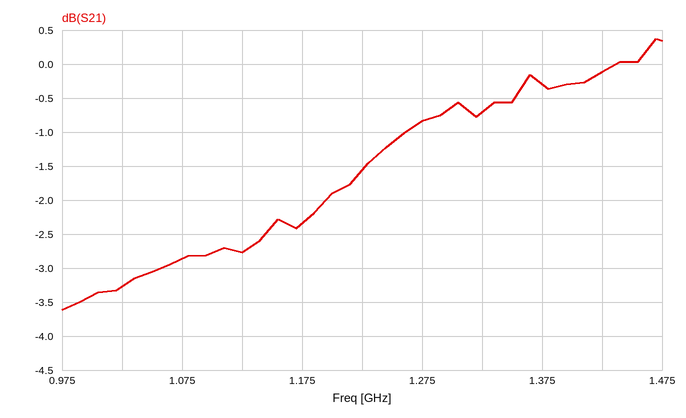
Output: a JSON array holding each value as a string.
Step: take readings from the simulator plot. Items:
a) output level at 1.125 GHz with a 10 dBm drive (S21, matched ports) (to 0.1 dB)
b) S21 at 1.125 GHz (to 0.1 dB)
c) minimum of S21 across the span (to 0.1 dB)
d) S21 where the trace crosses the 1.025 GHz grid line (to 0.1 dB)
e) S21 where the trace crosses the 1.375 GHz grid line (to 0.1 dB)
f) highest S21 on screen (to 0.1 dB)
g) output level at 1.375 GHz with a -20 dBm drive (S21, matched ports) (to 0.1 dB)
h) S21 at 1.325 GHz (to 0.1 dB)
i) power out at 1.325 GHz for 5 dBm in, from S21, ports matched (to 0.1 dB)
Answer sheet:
["7.2 dBm", "-2.8 dB", "-3.6 dB", "-3.3 dB", "-0.3 dB", "0.4 dB", "-20.3 dBm", "-0.7 dB", "4.3 dBm"]
